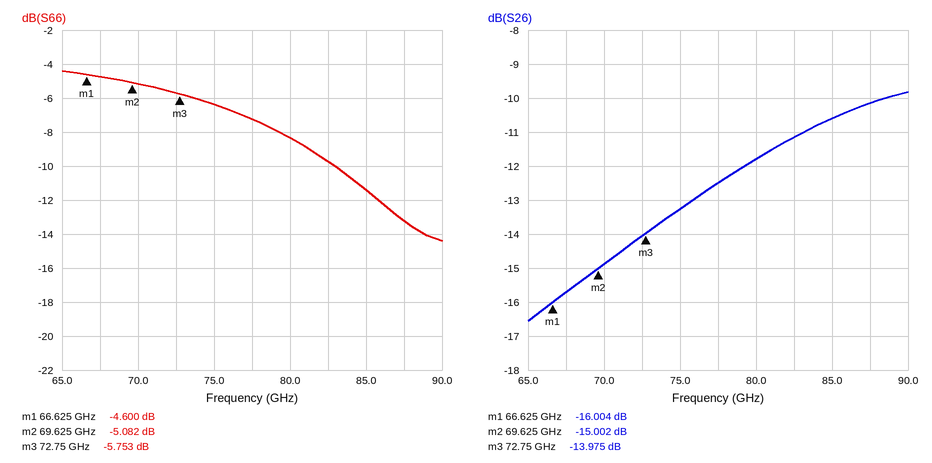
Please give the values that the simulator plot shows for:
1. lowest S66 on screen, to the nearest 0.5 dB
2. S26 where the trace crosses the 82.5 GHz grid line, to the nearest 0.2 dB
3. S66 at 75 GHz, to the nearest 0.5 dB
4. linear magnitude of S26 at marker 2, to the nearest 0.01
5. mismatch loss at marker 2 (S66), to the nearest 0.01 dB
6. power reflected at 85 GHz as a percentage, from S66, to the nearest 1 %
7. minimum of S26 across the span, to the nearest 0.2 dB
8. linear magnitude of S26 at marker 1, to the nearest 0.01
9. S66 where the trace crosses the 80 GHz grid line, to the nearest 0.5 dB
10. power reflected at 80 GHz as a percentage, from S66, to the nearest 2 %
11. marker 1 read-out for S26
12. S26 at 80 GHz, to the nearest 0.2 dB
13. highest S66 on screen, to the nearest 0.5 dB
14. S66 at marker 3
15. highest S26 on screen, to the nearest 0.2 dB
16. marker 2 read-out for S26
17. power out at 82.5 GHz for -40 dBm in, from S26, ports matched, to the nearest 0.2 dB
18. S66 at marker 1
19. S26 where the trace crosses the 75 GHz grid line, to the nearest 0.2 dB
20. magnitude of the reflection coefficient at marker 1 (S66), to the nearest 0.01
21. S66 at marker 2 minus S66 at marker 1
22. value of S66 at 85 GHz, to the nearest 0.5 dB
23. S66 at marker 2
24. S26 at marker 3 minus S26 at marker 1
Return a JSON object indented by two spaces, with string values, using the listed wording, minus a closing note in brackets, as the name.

{
  "lowest S66 on screen, to the nearest 0.5 dB": "-14.5 dB",
  "S26 where the trace crosses the 82.5 GHz grid line, to the nearest 0.2 dB": "-11.2 dB",
  "S66 at 75 GHz, to the nearest 0.5 dB": "-6.5 dB",
  "linear magnitude of S26 at marker 2, to the nearest 0.01": "0.18",
  "mismatch loss at marker 2 (S66), to the nearest 0.01 dB": "1.61 dB",
  "power reflected at 85 GHz as a percentage, from S66, to the nearest 1 %": "7 %",
  "minimum of S26 across the span, to the nearest 0.2 dB": "-16.6 dB",
  "linear magnitude of S26 at marker 1, to the nearest 0.01": "0.16",
  "S66 where the trace crosses the 80 GHz grid line, to the nearest 0.5 dB": "-8.5 dB",
  "power reflected at 80 GHz as a percentage, from S66, to the nearest 2 %": "14 %",
  "marker 1 read-out for S26": "-16.004 dB",
  "S26 at 80 GHz, to the nearest 0.2 dB": "-11.8 dB",
  "highest S66 on screen, to the nearest 0.5 dB": "-4.5 dB",
  "S66 at marker 3": "-5.753 dB",
  "highest S26 on screen, to the nearest 0.2 dB": "-9.8 dB",
  "marker 2 read-out for S26": "-15.002 dB",
  "power out at 82.5 GHz for -40 dBm in, from S26, ports matched, to the nearest 0.2 dB": "-51.2 dBm",
  "S66 at marker 1": "-4.600 dB",
  "S26 where the trace crosses the 75 GHz grid line, to the nearest 0.2 dB": "-13.2 dB",
  "magnitude of the reflection coefficient at marker 1 (S66), to the nearest 0.01": "0.59",
  "S66 at marker 2 minus S66 at marker 1": "-0.482 dB",
  "value of S66 at 85 GHz, to the nearest 0.5 dB": "-11.5 dB",
  "S66 at marker 2": "-5.082 dB",
  "S26 at marker 3 minus S26 at marker 1": "2.029 dB"
}
